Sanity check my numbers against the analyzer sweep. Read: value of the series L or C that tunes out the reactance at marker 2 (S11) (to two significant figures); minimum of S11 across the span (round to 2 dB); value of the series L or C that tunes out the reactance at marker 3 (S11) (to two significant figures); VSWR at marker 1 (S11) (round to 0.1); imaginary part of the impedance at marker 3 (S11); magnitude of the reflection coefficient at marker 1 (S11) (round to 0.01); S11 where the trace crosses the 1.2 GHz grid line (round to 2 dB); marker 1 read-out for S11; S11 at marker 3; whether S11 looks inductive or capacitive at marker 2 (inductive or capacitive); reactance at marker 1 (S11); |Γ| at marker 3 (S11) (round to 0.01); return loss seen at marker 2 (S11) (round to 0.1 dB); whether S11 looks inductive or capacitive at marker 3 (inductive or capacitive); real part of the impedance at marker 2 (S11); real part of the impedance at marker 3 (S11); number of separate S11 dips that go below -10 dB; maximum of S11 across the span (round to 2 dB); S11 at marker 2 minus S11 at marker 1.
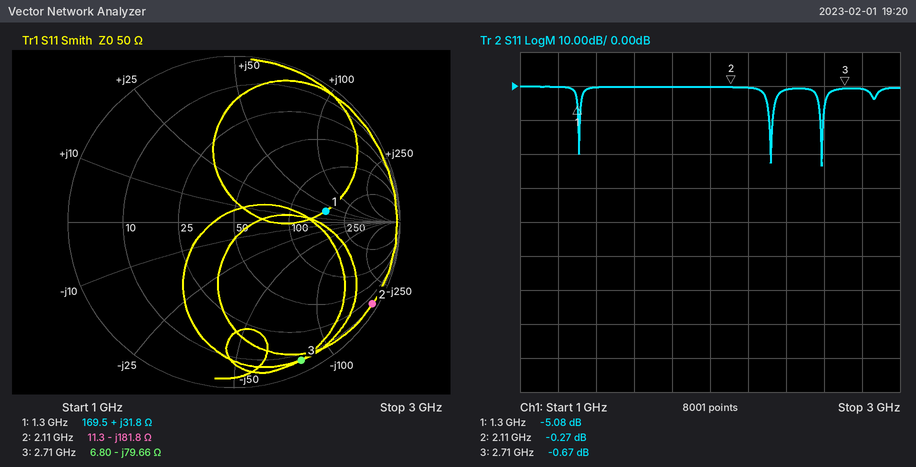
14 nH
-24 dB
4.7 nH
3.5
-79.66 Ω
0.56
0 dB
-5.08 dB
-0.67 dB
capacitive
+31.8 Ω
0.93
0.3 dB
capacitive
11.3 Ω
6.80 Ω
3
0 dB
4.81 dB
